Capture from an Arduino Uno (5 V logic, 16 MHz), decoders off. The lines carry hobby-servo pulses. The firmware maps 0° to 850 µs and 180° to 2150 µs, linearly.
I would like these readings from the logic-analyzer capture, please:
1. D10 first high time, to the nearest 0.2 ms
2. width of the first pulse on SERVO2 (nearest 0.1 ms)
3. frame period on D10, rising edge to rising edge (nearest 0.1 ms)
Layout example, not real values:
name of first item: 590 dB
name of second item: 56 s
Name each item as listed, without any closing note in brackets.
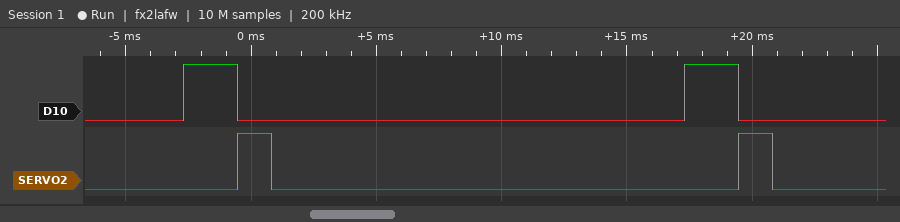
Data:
D10 first high time, to the nearest 0.2 ms: 2.2 ms
width of the first pulse on SERVO2: 1.4 ms
frame period on D10, rising edge to rising edge: 20.0 ms
